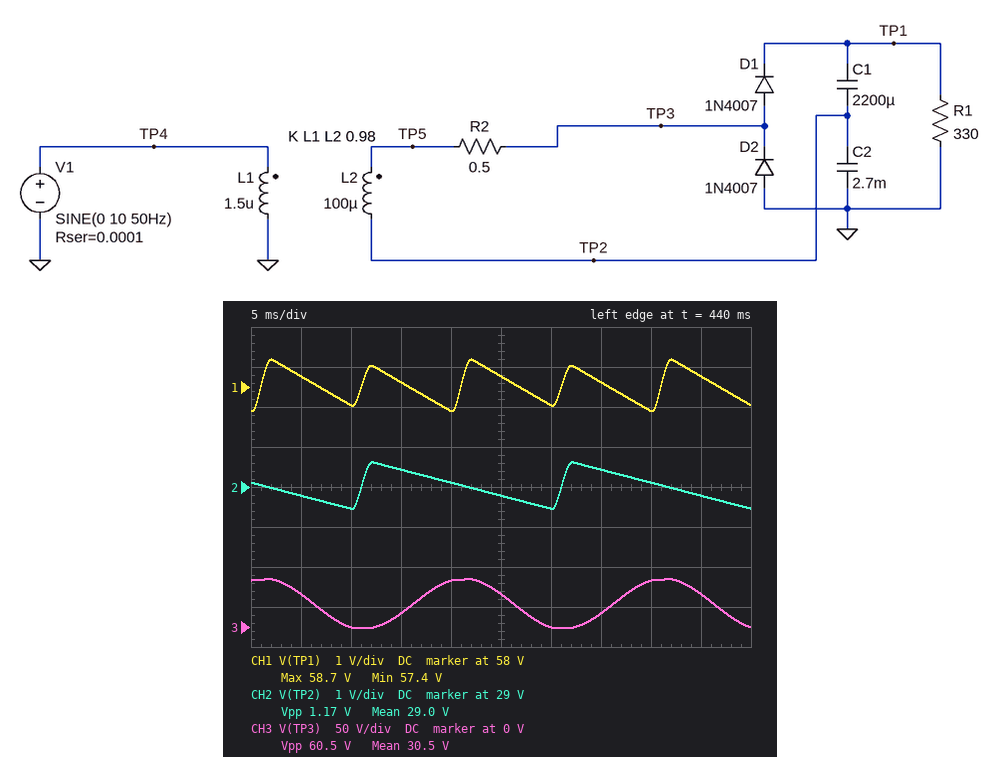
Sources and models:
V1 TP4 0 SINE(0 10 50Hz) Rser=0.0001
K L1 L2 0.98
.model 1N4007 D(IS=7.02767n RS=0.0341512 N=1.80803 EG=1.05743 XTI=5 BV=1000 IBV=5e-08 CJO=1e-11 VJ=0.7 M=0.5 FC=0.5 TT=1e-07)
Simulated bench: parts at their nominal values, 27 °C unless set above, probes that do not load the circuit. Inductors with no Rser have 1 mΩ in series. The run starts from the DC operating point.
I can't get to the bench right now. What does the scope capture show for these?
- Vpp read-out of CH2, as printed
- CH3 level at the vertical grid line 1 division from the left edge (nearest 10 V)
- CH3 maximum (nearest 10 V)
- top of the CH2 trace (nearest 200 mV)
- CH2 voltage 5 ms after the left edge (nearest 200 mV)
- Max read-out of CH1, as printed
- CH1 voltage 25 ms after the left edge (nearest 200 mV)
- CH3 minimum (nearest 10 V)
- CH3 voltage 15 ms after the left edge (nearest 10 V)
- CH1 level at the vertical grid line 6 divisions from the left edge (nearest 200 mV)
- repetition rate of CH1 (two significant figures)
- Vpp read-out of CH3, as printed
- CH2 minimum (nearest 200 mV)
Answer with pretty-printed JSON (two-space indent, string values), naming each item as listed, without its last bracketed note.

{
  "Vpp read-out of CH2, as printed": "1.17 V",
  "CH3 level at the vertical grid line 1 division from the left edge": "40 V",
  "CH3 maximum": "60 V",
  "top of the CH2 trace": "29.6 V",
  "CH2 voltage 5 ms after the left edge": "28.8 V",
  "Max read-out of CH1, as printed": "58.7 V",
  "CH1 voltage 25 ms after the left edge": "58.2 V",
  "CH3 minimum": "0 V",
  "CH3 voltage 15 ms after the left edge": "20 V",
  "CH1 level at the vertical grid line 6 divisions from the left edge": "57.6 V",
  "repetition rate of CH1": "100 Hz",
  "Vpp read-out of CH3, as printed": "60.5 V",
  "CH2 minimum": "28.4 V"
}
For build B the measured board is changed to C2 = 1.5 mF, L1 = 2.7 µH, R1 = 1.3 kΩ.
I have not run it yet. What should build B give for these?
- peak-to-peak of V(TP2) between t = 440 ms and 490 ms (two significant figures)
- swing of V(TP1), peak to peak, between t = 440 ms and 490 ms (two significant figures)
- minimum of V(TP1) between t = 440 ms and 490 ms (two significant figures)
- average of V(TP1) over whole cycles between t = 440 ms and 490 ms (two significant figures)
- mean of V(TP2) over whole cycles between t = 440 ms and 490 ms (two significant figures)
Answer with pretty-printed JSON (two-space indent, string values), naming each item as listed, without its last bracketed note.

{
  "peak-to-peak of V(TP2) between t = 440 ms and 490 ms": "660 mV",
  "swing of V(TP1), peak to peak, between t = 440 ms and 490 ms": "630 mV",
  "minimum of V(TP1) between t = 440 ms and 490 ms": "69 V",
  "average of V(TP1) over whole cycles between t = 440 ms and 490 ms": "70 V",
  "mean of V(TP2) over whole cycles between t = 440 ms and 490 ms": "35 V"
}
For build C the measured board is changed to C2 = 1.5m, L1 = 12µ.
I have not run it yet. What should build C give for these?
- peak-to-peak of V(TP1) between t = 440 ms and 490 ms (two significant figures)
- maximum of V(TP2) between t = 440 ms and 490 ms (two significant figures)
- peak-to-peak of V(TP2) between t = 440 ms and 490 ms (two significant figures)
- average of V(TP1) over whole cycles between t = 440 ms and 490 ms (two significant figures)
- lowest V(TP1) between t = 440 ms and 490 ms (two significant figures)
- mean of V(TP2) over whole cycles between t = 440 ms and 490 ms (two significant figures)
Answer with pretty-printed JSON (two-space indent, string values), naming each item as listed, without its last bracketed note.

{
  "peak-to-peak of V(TP1) between t = 440 ms and 490 ms": "1.7 V",
  "maximum of V(TP2) between t = 440 ms and 490 ms": "26 V",
  "peak-to-peak of V(TP2) between t = 440 ms and 490 ms": "1.8 V",
  "average of V(TP1) over whole cycles between t = 440 ms and 490 ms": "50 V",
  "lowest V(TP1) between t = 440 ms and 490 ms": "49 V",
  "mean of V(TP2) over whole cycles between t = 440 ms and 490 ms": "25 V"
}
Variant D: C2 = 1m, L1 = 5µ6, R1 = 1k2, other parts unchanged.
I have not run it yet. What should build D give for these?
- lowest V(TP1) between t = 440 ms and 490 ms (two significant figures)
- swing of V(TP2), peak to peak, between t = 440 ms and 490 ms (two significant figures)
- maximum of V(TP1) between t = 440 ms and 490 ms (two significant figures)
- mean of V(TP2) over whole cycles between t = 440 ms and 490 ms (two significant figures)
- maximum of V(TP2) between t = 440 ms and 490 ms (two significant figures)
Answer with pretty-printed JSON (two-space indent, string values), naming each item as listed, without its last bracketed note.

{
  "lowest V(TP1) between t = 440 ms and 490 ms": "66 V",
  "swing of V(TP2), peak to peak, between t = 440 ms and 490 ms": "1.0 V",
  "maximum of V(TP1) between t = 440 ms and 490 ms": "67 V",
  "mean of V(TP2) over whole cycles between t = 440 ms and 490 ms": "33 V",
  "maximum of V(TP2) between t = 440 ms and 490 ms": "34 V"
}
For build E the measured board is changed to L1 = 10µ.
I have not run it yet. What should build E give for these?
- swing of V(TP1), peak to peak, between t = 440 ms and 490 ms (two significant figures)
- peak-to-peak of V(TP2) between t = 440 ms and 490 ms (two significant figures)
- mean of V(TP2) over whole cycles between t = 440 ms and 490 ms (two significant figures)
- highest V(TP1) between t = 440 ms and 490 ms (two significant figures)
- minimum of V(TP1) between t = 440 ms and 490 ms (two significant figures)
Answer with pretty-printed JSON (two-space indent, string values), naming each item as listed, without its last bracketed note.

{
  "swing of V(TP1), peak to peak, between t = 440 ms and 490 ms": "1.2 V",
  "peak-to-peak of V(TP2) between t = 440 ms and 490 ms": "1.1 V",
  "mean of V(TP2) over whole cycles between t = 440 ms and 490 ms": "27 V",
  "highest V(TP1) between t = 440 ms and 490 ms": "54 V",
  "minimum of V(TP1) between t = 440 ms and 490 ms": "53 V"
}
